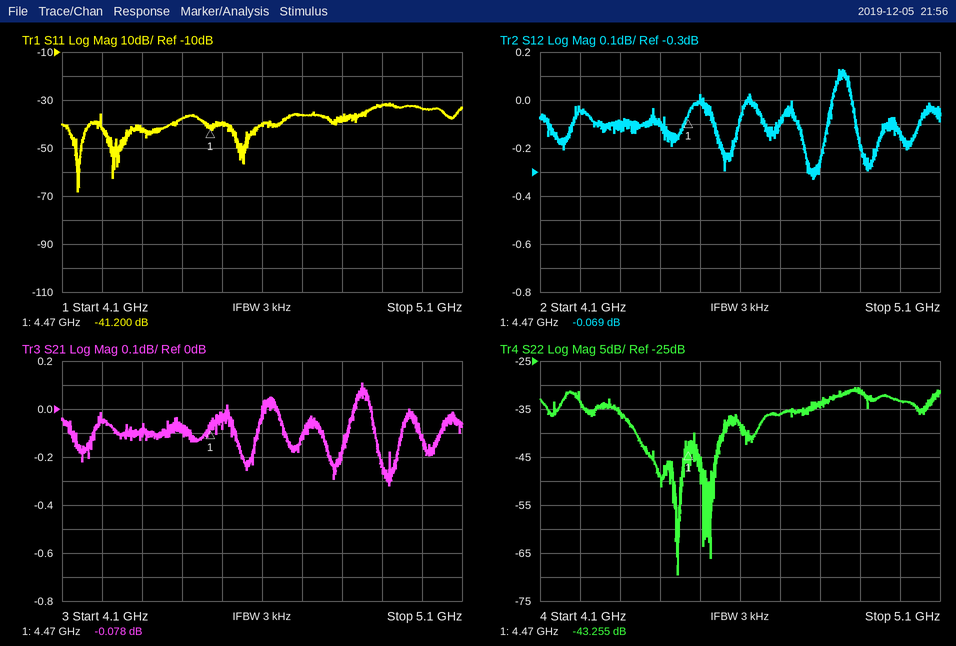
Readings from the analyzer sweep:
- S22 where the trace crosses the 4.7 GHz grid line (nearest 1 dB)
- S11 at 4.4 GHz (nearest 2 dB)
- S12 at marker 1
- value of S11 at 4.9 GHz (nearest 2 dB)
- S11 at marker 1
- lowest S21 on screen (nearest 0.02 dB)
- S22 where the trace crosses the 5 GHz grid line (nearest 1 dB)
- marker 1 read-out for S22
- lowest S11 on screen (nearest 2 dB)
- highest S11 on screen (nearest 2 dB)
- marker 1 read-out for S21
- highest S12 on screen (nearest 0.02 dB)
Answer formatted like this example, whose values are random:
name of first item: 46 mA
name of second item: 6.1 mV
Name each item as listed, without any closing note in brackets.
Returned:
S22 where the trace crosses the 4.7 GHz grid line: -36 dB
S11 at 4.4 GHz: -38 dB
S12 at marker 1: -0.069 dB
value of S11 at 4.9 GHz: -32 dB
S11 at marker 1: -41.200 dB
lowest S21 on screen: -0.32 dB
S22 where the trace crosses the 5 GHz grid line: -33 dB
marker 1 read-out for S22: -43.255 dB
lowest S11 on screen: -68 dB
highest S11 on screen: -32 dB
marker 1 read-out for S21: -0.078 dB
highest S12 on screen: 0.12 dB
